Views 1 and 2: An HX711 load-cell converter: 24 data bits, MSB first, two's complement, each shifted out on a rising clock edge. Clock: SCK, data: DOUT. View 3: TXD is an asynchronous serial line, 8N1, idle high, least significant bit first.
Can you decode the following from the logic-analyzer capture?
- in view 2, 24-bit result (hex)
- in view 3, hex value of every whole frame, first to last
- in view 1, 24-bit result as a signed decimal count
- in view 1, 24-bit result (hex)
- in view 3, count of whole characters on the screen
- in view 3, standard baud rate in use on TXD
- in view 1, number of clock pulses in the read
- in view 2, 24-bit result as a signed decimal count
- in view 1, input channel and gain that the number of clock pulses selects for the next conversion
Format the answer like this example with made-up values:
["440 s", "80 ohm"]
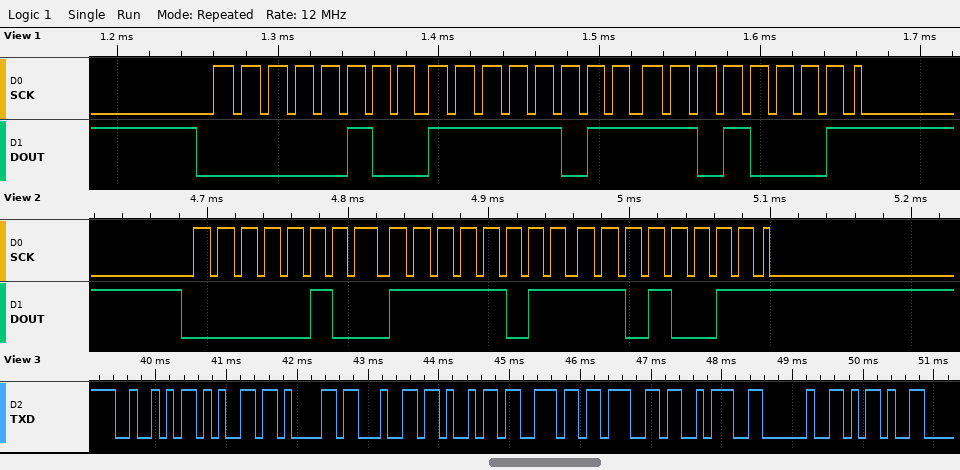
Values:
["0x04FBD3", "0x52 0x65 0x61 0x64 0x69 0x6E 0x67 0x3A 0x20 0x2D", "326609", "0x04FBD1", "10", "9600 baud", "25", "326611", "channel A, gain 128"]
